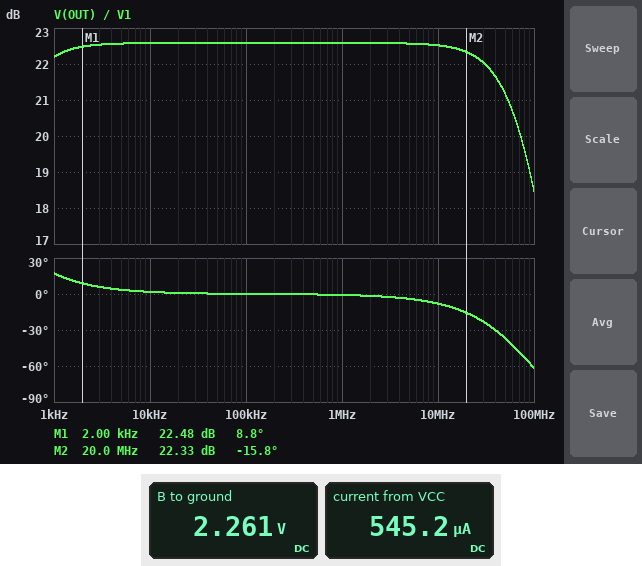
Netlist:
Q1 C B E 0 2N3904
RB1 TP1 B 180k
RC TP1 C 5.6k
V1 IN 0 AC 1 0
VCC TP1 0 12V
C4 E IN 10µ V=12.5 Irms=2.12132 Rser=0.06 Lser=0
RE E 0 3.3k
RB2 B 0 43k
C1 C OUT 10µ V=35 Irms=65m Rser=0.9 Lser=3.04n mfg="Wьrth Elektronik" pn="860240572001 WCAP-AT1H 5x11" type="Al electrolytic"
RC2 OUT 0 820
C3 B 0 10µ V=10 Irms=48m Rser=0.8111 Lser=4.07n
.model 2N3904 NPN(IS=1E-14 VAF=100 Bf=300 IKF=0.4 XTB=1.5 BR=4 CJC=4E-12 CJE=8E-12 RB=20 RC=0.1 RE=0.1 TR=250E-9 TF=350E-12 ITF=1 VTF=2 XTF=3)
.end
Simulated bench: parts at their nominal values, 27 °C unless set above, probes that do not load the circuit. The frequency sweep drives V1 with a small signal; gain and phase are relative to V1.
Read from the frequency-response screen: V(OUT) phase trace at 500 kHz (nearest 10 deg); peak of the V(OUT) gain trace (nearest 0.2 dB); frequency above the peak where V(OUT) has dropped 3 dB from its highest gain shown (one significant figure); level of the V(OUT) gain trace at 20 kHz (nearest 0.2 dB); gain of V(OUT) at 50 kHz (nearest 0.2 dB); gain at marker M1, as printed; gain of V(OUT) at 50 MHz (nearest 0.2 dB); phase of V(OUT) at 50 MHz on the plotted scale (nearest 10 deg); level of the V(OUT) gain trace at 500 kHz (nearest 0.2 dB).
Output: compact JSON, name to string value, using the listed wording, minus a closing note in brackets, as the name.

{"V(OUT) phase trace at 500 kHz": "0 deg", "peak of the V(OUT) gain trace": "22.6 dB", "frequency above the peak where V(OUT) has dropped 3 dB from its highest gain shown": "80 MHz", "level of the V(OUT) gain trace at 20 kHz": "22.6 dB", "gain of V(OUT) at 50 kHz": "22.6 dB", "gain at marker M1, as printed": "22.48 dB", "gain of V(OUT) at 50 MHz": "21.2 dB", "phase of V(OUT) at 50 MHz on the plotted scale": "-40 deg", "level of the V(OUT) gain trace at 500 kHz": "22.6 dB"}
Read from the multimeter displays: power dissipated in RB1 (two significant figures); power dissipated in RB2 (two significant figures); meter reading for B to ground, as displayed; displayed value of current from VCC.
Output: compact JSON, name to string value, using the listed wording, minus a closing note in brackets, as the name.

{"power dissipated in RB1": "530 µW", "power dissipated in RB2": "120 µW", "meter reading for B to ground, as displayed": "2.261 V", "displayed value of current from VCC": "545.2 µA"}
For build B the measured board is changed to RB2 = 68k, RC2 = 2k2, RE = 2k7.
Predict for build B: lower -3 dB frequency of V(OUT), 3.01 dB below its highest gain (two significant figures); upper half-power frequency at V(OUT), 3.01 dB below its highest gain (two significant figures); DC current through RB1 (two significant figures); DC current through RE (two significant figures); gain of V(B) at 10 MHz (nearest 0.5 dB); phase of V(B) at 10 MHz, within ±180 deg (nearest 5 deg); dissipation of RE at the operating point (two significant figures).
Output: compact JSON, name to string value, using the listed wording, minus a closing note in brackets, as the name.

{"lower -3 dB frequency of V(OUT), 3.01 dB below its highest gain": "560 Hz", "upper half-power frequency at V(OUT), 3.01 dB below its highest gain": "26 MHz", "DC current through RB1": "49 µA", "DC current through RE": "920 µA", "gain of V(B) at 10 MHz": "-42.5 dB", "phase of V(B) at 10 MHz, within ±180 deg": "85 deg", "dissipation of RE at the operating point": "2.3 mW"}
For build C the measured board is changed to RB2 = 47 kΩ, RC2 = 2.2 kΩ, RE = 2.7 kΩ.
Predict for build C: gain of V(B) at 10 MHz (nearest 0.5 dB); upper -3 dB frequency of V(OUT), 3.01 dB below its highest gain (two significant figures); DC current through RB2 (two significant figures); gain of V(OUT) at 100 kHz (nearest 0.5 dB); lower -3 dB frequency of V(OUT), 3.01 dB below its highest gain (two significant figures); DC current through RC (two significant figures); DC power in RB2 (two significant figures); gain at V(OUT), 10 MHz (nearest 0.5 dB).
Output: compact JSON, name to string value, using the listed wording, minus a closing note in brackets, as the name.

{"gain of V(B) at 10 MHz": "-46.0 dB", "upper -3 dB frequency of V(OUT), 3.01 dB below its highest gain": "33 MHz", "DC current through RB2": "51 µA", "gain of V(OUT) at 100 kHz": "32.0 dB", "lower -3 dB frequency of V(OUT), 3.01 dB below its highest gain": "400 Hz", "DC current through RC": "650 µA", "DC power in RB2": "120 µW", "gain at V(OUT), 10 MHz": "31.5 dB"}
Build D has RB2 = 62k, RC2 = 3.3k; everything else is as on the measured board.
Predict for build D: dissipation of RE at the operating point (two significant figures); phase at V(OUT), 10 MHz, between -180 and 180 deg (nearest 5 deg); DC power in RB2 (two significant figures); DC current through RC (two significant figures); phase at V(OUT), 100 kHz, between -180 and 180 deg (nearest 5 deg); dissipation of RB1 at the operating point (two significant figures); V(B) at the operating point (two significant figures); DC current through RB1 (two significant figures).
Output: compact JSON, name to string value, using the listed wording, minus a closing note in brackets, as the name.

{"dissipation of RE at the operating point": "1.6 mW", "phase at V(OUT), 10 MHz, between -180 and 180 deg": "-25 deg", "DC power in RB2": "140 µW", "DC current through RC": "700 µA", "phase at V(OUT), 100 kHz, between -180 and 180 deg": "0 deg", "dissipation of RB1 at the operating point": "450 µW", "V(B) at the operating point": "3.0 V", "DC current through RB1": "50 µA"}
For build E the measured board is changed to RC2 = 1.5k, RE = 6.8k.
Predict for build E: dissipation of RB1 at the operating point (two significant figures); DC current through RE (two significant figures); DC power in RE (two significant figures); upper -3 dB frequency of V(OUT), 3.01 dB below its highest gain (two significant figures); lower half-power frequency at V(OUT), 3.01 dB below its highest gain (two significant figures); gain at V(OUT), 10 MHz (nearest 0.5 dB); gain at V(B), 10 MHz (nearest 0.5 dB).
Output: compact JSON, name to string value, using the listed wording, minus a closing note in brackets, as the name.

{"dissipation of RB1 at the operating point": "520 µW", "DC current through RE": "250 µA", "DC power in RE": "410 µW", "upper -3 dB frequency of V(OUT), 3.01 dB below its highest gain": "62 MHz", "lower half-power frequency at V(OUT), 3.01 dB below its highest gain": "150 Hz", "gain at V(OUT), 10 MHz": "21.0 dB", "gain at V(B), 10 MHz": "-54.5 dB"}
